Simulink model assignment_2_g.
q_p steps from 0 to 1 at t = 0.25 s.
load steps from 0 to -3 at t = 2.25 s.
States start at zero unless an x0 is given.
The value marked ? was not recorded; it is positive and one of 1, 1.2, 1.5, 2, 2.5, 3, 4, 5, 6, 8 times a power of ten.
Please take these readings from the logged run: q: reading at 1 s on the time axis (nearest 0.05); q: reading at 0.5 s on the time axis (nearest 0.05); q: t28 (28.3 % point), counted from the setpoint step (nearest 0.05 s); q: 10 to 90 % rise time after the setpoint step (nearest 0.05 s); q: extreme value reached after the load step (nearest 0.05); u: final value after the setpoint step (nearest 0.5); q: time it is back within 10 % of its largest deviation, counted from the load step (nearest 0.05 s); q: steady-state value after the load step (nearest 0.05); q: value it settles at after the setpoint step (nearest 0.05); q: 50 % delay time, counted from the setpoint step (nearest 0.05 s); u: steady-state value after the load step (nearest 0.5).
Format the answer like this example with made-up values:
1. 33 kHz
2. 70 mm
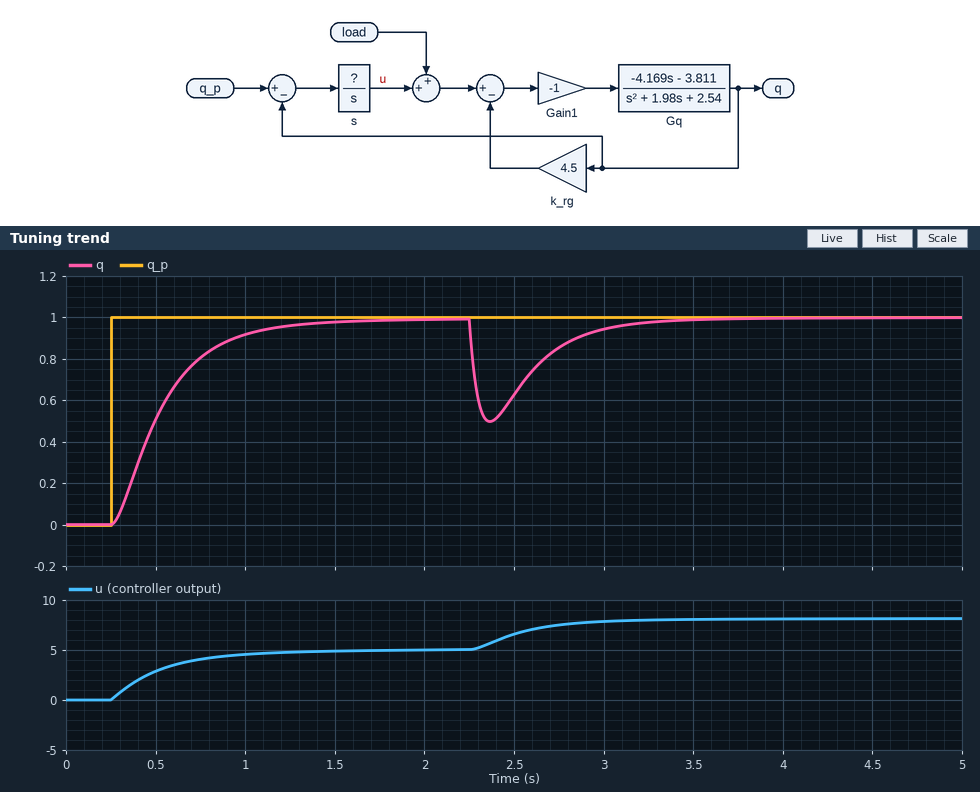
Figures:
1. 0.90
2. 0.50
3. 0.15 s
4. 0.60 s
5. 0.50
6. 5.0
7. 0.80 s
8. 1.00
9. 1.00
10. 0.25 s
11. 8.0
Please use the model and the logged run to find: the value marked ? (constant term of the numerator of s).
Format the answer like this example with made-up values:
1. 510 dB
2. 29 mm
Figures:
1. 15
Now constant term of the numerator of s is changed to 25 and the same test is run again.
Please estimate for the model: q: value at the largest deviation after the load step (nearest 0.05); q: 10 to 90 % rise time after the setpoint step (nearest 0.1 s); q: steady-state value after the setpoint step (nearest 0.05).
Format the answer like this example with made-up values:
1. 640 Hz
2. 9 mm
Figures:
1. 0.55
2. 0.3 s
3. 1.00
